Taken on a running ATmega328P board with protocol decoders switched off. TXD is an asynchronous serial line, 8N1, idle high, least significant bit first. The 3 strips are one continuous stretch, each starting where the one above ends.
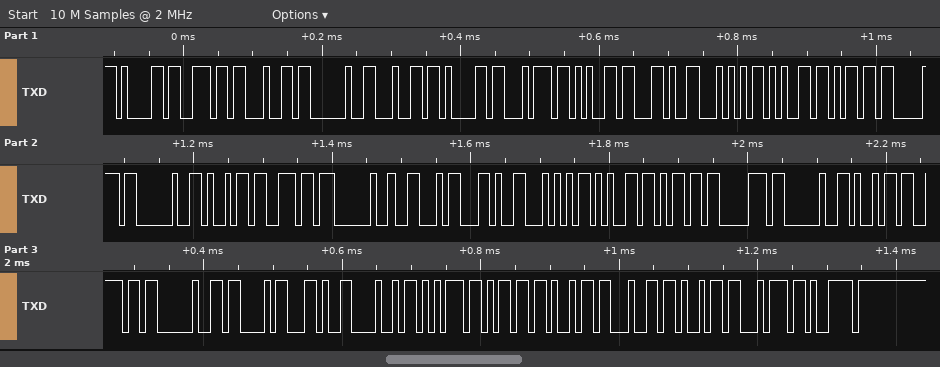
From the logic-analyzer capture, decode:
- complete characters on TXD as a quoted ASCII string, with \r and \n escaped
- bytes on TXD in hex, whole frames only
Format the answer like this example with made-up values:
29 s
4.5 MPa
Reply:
"and date,Temp in F,Temp in C,Humidity"
0x61 0x6E 0x64 0x20 0x64 0x61 0x74 0x65 0x2C 0x54 0x65 0x6D 0x70 0x20 0x69 0x6E 0x20 0x46 0x2C 0x54 0x65 0x6D 0x70 0x20 0x69 0x6E 0x20 0x43 0x2C 0x48 0x75 0x6D 0x69 0x64 0x69 0x74 0x79
